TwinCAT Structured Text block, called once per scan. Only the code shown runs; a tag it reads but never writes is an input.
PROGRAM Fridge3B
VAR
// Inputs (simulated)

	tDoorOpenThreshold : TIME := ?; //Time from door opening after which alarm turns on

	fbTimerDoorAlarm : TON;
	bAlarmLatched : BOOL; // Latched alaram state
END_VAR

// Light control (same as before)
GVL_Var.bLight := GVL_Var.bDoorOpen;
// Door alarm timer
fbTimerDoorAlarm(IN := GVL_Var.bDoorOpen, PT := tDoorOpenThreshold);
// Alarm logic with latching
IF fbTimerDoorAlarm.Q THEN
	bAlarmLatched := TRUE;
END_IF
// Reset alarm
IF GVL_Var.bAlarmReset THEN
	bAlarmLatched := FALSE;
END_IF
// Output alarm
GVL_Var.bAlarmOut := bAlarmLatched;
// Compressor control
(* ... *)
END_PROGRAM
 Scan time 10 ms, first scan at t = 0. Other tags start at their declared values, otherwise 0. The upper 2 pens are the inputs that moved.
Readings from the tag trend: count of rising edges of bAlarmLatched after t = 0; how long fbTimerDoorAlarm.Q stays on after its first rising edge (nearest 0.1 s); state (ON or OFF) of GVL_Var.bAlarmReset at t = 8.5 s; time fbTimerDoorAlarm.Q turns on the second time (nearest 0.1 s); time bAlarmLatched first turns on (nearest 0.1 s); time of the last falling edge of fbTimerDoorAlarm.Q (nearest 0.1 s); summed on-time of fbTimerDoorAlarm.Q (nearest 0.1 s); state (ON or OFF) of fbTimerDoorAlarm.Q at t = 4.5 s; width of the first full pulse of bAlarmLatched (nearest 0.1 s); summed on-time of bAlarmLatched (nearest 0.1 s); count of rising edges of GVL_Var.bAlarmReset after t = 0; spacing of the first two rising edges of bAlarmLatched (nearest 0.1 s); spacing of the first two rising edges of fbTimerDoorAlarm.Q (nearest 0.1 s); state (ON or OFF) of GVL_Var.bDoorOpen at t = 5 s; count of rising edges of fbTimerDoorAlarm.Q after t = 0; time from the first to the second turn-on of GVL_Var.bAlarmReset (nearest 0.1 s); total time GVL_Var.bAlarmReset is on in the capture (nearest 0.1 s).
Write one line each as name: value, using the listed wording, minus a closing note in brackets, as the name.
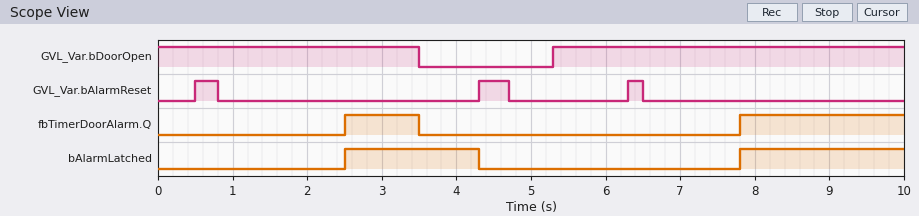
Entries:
count of rising edges of bAlarmLatched after t = 0: 2
how long fbTimerDoorAlarm.Q stays on after its first rising edge: 1.0 s
state (ON or OFF) of GVL_Var.bAlarmReset at t = 8.5 s: OFF
time fbTimerDoorAlarm.Q turns on the second time: 7.8 s
time bAlarmLatched first turns on: 2.5 s
time of the last falling edge of fbTimerDoorAlarm.Q: 3.5 s
summed on-time of fbTimerDoorAlarm.Q: 3.2 s
state (ON or OFF) of fbTimerDoorAlarm.Q at t = 4.5 s: OFF
width of the first full pulse of bAlarmLatched: 1.8 s
summed on-time of bAlarmLatched: 4.0 s
count of rising edges of GVL_Var.bAlarmReset after t = 0: 3
spacing of the first two rising edges of bAlarmLatched: 5.3 s
spacing of the first two rising edges of fbTimerDoorAlarm.Q: 5.3 s
state (ON or OFF) of GVL_Var.bDoorOpen at t = 5 s: OFF
count of rising edges of fbTimerDoorAlarm.Q after t = 0: 2
time from the first to the second turn-on of GVL_Var.bAlarmReset: 3.8 s
total time GVL_Var.bAlarmReset is on in the capture: 0.9 s
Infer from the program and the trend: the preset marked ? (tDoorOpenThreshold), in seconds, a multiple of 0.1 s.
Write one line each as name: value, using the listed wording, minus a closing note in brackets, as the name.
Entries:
the preset marked ? (tDoorOpenThreshold), in seconds, a multiple of 0.1 s: 2.5 s
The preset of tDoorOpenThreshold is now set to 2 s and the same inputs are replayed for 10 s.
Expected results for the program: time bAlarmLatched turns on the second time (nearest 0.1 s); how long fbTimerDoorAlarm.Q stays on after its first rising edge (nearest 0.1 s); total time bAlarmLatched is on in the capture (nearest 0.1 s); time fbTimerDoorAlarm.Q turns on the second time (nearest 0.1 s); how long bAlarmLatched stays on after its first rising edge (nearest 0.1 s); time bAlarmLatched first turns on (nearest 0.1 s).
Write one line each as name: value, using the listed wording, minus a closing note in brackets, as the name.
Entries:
time bAlarmLatched turns on the second time: 7.3 s
how long fbTimerDoorAlarm.Q stays on after its first rising edge: 1.5 s
total time bAlarmLatched is on in the capture: 5.0 s
time fbTimerDoorAlarm.Q turns on the second time: 7.3 s
how long bAlarmLatched stays on after its first rising edge: 2.3 s
time bAlarmLatched first turns on: 2.0 s
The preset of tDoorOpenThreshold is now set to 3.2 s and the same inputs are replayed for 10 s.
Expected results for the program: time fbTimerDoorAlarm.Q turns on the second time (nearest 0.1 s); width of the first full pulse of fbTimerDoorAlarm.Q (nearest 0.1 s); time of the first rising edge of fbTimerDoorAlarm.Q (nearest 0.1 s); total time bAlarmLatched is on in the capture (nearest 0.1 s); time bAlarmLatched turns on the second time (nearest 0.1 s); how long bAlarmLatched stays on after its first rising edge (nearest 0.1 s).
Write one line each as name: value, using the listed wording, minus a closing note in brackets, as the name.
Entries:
time fbTimerDoorAlarm.Q turns on the second time: 8.5 s
width of the first full pulse of fbTimerDoorAlarm.Q: 0.3 s
time of the first rising edge of fbTimerDoorAlarm.Q: 3.2 s
total time bAlarmLatched is on in the capture: 2.6 s
time bAlarmLatched turns on the second time: 8.5 s
how long bAlarmLatched stays on after its first rising edge: 1.1 s
